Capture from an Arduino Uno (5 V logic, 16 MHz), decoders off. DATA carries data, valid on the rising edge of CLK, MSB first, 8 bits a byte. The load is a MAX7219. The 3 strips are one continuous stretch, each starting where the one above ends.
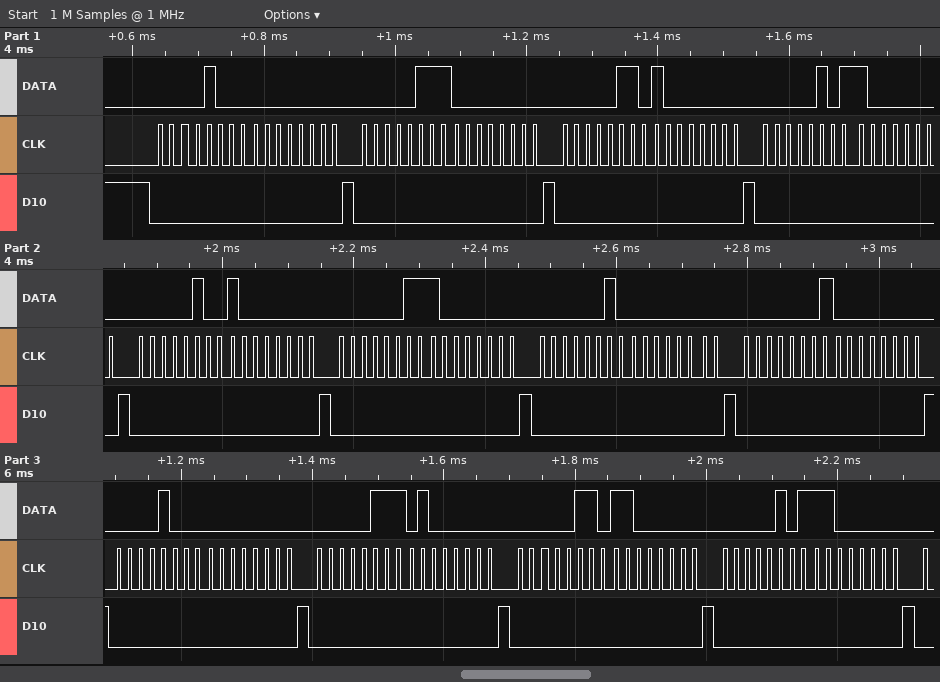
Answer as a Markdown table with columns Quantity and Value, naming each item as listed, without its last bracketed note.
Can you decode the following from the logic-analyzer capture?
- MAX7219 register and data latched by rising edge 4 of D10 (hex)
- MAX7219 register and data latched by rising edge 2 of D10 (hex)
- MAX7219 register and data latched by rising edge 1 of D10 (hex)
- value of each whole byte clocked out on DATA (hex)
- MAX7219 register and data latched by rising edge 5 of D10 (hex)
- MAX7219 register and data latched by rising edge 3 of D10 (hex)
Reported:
| Quantity | Value |
|---|---|
| MAX7219 register and data latched by rising edge 4 of D10 | register 0x5, data 0x80 |
| MAX7219 register and data latched by rising edge 2 of D10 | register 0x7, data 0x00 |
| MAX7219 register and data latched by rising edge 1 of D10 | register 0x8, data 0x00 |
| value of each whole byte clocked out on DATA | 08 00 07 00 06 80 05 80 04 80 03 80 02 00 01 00 08 00 07 40 06 C0 05 C0 |
| MAX7219 register and data latched by rising edge 5 of D10 | register 0x4, data 0x80 |
| MAX7219 register and data latched by rising edge 3 of D10 | register 0x6, data 0x80 |
